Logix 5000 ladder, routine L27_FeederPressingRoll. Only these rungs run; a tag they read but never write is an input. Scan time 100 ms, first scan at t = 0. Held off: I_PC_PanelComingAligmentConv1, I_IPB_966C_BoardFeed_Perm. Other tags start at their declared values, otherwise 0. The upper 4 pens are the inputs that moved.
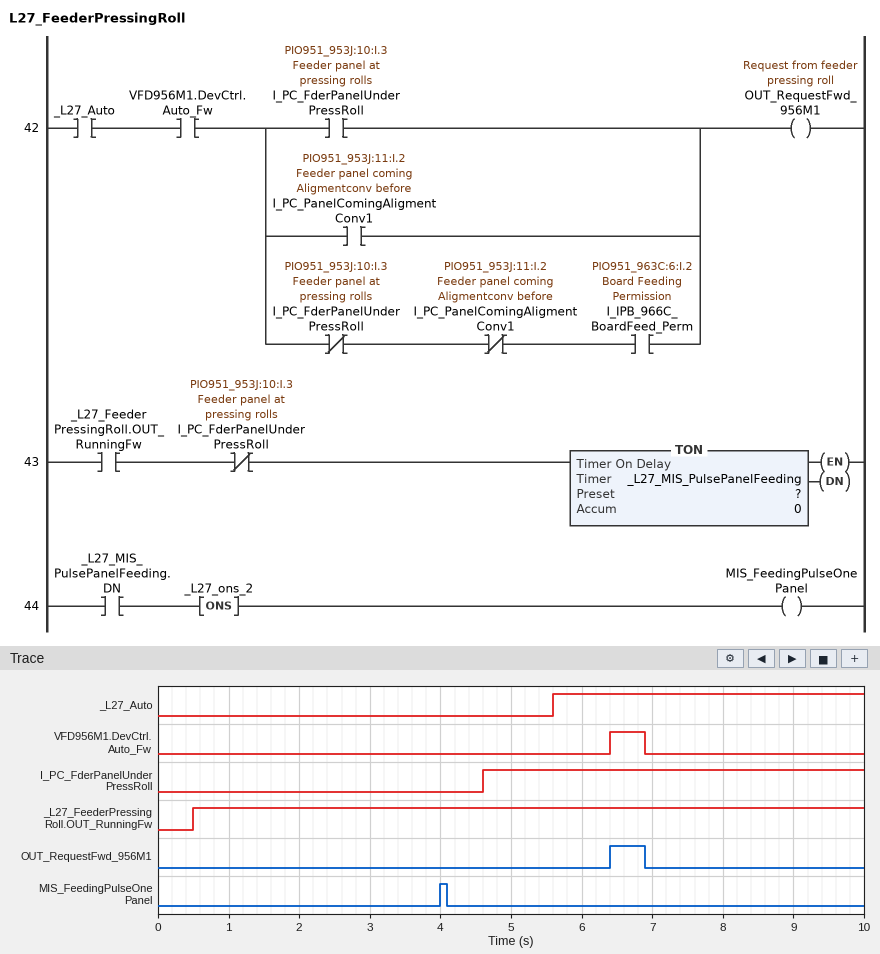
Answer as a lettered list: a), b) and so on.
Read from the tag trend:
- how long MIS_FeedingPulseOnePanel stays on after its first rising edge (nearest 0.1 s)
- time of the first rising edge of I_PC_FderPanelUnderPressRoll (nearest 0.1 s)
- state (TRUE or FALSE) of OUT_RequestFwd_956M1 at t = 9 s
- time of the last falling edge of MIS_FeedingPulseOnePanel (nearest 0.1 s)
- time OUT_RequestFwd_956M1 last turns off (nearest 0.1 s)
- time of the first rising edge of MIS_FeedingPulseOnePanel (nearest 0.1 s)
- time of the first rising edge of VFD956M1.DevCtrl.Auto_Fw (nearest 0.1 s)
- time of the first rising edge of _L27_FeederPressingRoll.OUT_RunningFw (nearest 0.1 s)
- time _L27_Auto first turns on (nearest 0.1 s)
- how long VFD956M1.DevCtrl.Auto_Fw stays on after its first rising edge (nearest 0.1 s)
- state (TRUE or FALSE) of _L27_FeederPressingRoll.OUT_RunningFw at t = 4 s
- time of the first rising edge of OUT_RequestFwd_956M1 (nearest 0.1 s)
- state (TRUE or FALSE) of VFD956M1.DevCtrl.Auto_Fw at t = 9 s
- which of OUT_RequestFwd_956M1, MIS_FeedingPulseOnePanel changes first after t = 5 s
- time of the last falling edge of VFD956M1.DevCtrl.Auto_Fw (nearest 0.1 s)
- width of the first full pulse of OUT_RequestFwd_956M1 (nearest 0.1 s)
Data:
a) 0.1 s
b) 4.6 s
c) FALSE
d) 4.1 s
e) 6.9 s
f) 4.0 s
g) 6.4 s
h) 0.5 s
i) 5.6 s
j) 0.5 s
k) TRUE
l) 6.4 s
m) FALSE
n) OUT_RequestFwd_956M1
o) 6.9 s
p) 0.5 s
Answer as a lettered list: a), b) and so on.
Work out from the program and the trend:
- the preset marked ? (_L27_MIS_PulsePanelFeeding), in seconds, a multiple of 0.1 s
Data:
a) 3.5 s
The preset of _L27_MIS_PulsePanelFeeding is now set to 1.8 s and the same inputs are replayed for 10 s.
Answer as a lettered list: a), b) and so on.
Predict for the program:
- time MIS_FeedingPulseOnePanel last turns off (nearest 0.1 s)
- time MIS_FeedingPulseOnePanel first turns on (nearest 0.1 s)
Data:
a) 2.4 s
b) 2.3 s
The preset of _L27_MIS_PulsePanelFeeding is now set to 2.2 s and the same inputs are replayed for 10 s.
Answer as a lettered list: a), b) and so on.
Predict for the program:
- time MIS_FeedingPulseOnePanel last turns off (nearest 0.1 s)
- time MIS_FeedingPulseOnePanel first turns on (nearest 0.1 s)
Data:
a) 2.8 s
b) 2.7 s
